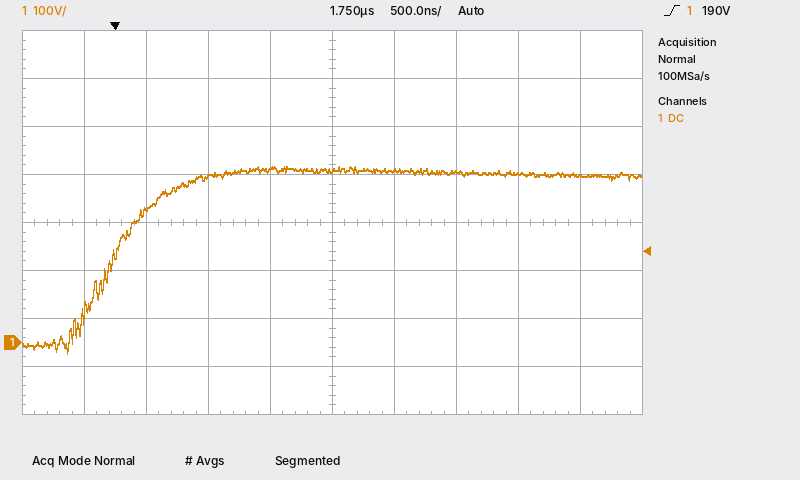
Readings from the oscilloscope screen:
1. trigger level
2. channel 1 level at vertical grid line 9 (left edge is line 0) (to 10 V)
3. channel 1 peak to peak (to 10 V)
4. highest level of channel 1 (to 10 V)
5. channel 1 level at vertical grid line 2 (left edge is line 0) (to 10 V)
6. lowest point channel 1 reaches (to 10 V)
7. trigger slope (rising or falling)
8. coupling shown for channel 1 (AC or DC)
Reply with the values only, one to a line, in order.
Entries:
190 V
350 V
390 V
370 V
270 V
-20 V
rising
DC
